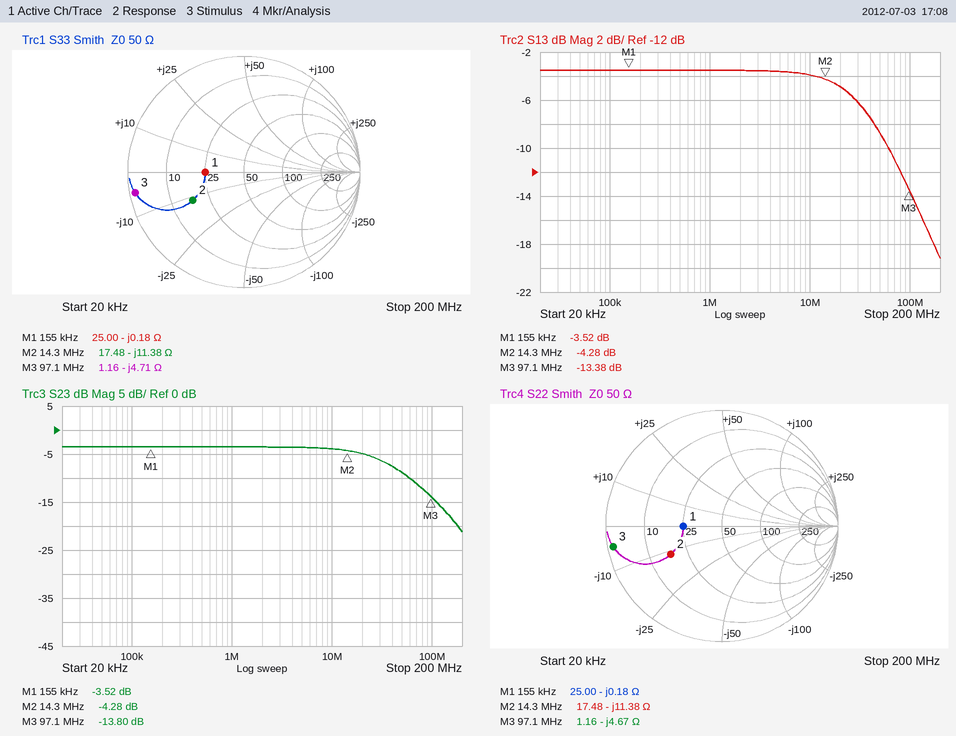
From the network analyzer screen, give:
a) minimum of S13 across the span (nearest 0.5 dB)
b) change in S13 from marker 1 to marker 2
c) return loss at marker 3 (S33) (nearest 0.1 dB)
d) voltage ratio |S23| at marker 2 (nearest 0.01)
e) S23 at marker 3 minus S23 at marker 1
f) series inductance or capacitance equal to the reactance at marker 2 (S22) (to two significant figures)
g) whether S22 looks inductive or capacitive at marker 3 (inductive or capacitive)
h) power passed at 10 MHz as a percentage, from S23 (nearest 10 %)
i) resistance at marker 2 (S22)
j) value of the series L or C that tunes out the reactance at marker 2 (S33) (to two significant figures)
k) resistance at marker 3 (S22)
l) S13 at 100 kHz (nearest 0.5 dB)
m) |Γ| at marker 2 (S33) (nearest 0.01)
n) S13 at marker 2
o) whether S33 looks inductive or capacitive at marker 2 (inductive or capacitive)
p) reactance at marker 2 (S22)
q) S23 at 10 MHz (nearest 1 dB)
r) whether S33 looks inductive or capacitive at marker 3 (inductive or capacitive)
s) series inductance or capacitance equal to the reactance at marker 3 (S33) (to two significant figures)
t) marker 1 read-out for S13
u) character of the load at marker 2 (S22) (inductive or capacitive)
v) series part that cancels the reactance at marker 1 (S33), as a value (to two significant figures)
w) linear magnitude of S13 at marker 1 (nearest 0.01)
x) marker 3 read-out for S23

-19.0 dB
-0.76 dB
0.4 dB
0.61
-10.28 dB
980 pF
capacitive
40 %
17.48 Ω
130 nH
1.16 Ω
-3.5 dB
0.50
-4.28 dB
capacitive
-11.38 Ω
-4 dB
capacitive
350 pF
-3.52 dB
capacitive
180 nH
0.67
-13.80 dB
